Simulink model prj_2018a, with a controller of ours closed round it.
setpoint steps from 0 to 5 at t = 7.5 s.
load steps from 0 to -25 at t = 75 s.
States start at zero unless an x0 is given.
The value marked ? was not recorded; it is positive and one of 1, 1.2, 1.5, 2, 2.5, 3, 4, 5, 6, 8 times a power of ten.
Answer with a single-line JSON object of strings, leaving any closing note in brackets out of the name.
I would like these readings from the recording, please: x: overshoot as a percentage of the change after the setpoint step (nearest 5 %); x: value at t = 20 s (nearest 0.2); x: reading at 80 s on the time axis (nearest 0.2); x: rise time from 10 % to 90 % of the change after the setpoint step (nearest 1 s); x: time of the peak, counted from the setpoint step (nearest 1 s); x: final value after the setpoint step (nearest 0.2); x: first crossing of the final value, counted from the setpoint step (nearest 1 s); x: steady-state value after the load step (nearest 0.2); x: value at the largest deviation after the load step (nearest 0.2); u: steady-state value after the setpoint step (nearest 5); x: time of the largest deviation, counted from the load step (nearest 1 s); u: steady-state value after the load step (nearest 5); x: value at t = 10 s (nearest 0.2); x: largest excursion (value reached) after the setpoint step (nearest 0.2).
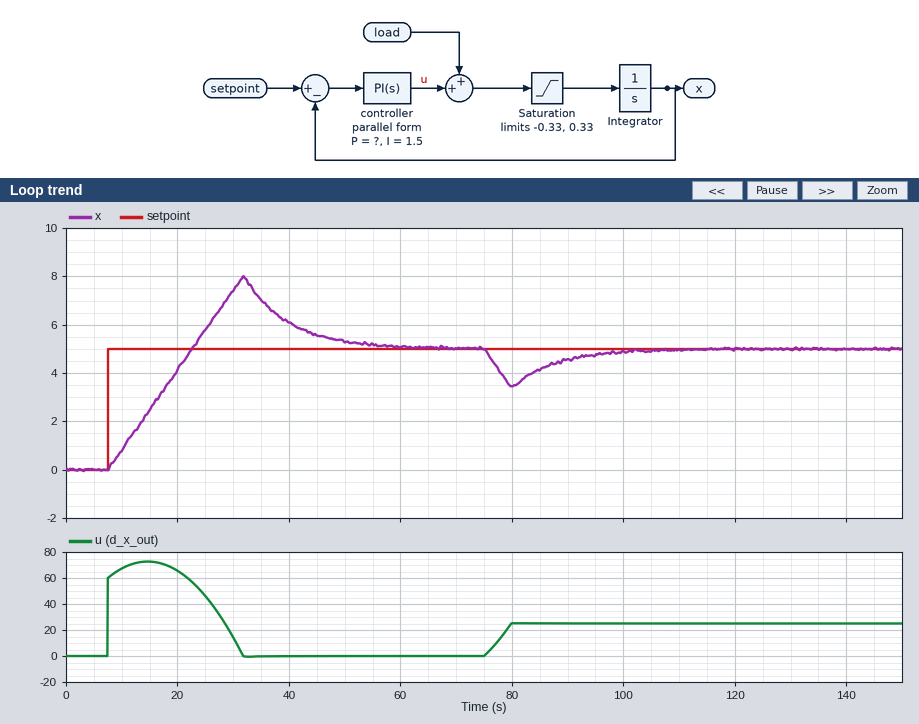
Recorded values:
{"x: overshoot as a percentage of the change after the setpoint step": "60 %", "x: value at t = 20 s": "4.2", "x: reading at 80 s on the time axis": "3.4", "x: rise time from 10 % to 90 % of the change after the setpoint step": "12 s", "x: time of the peak, counted from the setpoint step": "24 s", "x: final value after the setpoint step": "5.0", "x: first crossing of the final value, counted from the setpoint step": "15 s", "x: steady-state value after the load step": "5.0", "x: value at the largest deviation after the load step": "3.4", "u: steady-state value after the setpoint step": "0", "x: time of the largest deviation, counted from the load step": "5 s", "u: steady-state value after the load step": "25", "x: value at t = 10 s": "0.8", "x: largest excursion (value reached) after the setpoint step": "8.0"}
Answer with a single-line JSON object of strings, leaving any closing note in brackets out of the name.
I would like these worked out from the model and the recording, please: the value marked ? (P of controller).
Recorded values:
{"the value marked ?": "12"}
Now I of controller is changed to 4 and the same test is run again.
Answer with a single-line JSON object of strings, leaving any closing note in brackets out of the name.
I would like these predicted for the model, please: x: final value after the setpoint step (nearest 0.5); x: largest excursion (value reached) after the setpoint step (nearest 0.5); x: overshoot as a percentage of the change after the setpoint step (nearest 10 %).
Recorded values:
{"x: final value after the setpoint step": "5.0", "x: largest excursion (value reached) after the setpoint step": "9.0", "x: overshoot as a percentage of the change after the setpoint step": "80 %"}
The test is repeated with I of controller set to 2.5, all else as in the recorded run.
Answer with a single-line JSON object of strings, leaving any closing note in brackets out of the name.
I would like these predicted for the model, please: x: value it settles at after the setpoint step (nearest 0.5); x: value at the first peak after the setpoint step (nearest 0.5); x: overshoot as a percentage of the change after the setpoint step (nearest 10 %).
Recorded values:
{"x: value it settles at after the setpoint step": "5.0", "x: value at the first peak after the setpoint step": "8.5", "x: overshoot as a percentage of the change after the setpoint step": "70 %"}
